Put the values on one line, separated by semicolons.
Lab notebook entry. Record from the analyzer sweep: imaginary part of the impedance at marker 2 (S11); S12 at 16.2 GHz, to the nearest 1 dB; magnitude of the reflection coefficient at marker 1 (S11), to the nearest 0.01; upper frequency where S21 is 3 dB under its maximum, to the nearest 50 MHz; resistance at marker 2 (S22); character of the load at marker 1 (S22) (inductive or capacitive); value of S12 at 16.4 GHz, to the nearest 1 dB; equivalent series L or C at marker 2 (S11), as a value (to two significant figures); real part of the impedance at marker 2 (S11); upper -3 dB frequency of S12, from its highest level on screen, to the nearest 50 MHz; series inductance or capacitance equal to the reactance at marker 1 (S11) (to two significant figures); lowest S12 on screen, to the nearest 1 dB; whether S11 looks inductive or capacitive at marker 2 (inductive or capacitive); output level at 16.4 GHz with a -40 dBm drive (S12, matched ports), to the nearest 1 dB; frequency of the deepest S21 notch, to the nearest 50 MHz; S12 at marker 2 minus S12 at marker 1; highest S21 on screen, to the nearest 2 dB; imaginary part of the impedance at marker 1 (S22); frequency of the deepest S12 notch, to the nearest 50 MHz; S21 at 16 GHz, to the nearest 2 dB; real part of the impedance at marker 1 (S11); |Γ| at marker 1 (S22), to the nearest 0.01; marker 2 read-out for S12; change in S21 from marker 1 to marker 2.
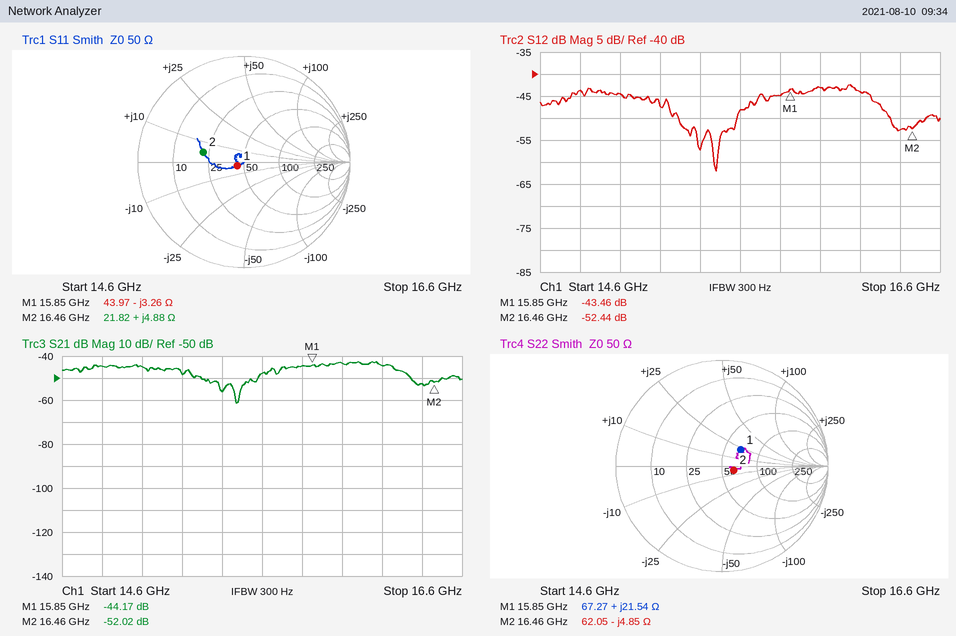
+4.88 Ω; -44 dB; 0.07; 16.25 GHz; 62.05 Ω; inductive; -53 dB; 47 pH; 21.82 Ω; 16.25 GHz; 3.1 pF; -62 dB; inductive; -93 dBm; 15.45 GHz; -8.98 dB; -42 dB; +21.54 Ω; 15.50 GHz; -44 dB; 43.97 Ω; 0.23; -52.44 dB; -7.85 dB
